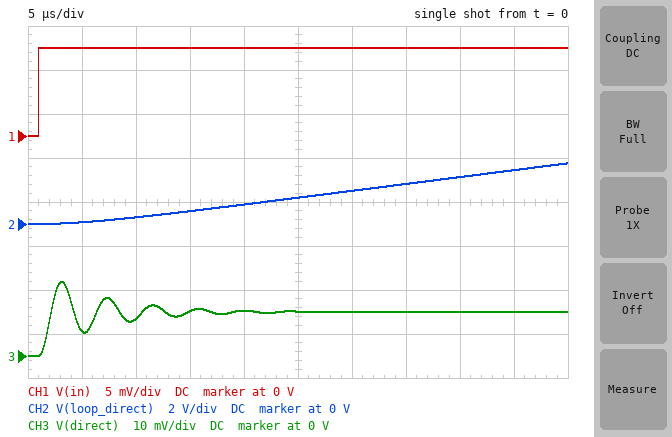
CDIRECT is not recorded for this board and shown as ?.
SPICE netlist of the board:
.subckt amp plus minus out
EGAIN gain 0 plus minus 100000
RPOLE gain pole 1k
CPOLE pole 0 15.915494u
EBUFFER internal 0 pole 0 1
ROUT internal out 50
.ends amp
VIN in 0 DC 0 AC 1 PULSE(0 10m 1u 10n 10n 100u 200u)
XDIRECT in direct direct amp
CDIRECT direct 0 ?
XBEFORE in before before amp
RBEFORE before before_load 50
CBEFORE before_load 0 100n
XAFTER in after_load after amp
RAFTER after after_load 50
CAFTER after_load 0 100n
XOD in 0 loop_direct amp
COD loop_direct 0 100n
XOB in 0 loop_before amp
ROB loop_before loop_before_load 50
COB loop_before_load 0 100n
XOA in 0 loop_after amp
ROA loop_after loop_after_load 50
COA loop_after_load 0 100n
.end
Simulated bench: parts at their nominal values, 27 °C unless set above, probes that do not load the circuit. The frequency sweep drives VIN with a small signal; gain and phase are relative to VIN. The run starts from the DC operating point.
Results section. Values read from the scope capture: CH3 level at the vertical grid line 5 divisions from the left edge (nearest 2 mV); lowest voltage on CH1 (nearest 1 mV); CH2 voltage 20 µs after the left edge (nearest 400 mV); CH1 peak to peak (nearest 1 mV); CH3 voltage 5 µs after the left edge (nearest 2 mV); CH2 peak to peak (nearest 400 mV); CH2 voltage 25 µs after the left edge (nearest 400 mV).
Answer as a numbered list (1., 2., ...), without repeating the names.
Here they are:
1. 10 mV
2. 0 V
3. 800 mV
4. 10 mV
5. 6 mV
6. 2.8 V
7. 1.2 V
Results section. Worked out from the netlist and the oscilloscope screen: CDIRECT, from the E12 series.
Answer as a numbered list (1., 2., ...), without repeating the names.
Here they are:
1. 56 nF
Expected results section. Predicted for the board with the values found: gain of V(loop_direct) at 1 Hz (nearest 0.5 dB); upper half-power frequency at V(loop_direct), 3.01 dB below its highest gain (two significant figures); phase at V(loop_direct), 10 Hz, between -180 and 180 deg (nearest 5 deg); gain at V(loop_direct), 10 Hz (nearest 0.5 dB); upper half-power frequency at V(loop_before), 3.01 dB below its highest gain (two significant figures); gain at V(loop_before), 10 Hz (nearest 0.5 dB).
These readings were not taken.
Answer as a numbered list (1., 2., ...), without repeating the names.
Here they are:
1. 100.0 dB
2. 10 Hz
3. -45 deg
4. 97.0 dB
5. 10 Hz
6. 97.0 dB
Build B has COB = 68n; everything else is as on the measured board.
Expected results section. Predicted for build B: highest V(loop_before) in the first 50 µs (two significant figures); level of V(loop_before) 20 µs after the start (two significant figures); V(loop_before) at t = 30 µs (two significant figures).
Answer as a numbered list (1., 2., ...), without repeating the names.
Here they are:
1. 2.9 V
2. 990 mV
3. 1.6 V
